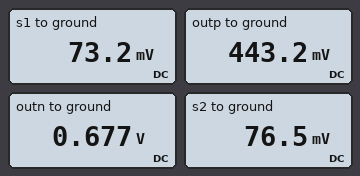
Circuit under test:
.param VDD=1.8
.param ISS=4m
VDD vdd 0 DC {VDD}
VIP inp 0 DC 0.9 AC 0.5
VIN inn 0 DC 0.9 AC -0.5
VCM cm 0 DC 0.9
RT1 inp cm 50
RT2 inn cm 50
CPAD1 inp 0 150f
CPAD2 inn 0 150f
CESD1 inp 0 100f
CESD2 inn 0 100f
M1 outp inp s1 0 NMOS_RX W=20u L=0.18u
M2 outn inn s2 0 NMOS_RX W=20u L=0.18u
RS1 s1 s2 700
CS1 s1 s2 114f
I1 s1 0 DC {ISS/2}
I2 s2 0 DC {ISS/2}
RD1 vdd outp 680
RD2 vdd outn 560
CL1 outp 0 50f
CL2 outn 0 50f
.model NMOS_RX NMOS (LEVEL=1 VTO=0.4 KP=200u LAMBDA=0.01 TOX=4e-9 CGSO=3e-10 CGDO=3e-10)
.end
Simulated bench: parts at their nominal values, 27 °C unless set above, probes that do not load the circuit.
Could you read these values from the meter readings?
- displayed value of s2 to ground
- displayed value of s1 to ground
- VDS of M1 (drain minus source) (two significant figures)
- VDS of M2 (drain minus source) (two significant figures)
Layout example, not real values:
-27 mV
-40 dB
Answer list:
76.5 mV
73.2 mV
370 mV
600 mV
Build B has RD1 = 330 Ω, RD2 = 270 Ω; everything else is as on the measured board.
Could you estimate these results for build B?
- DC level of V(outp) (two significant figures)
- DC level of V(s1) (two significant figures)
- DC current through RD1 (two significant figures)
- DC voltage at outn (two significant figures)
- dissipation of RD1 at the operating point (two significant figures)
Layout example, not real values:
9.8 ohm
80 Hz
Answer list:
1.1 V
78 mV
2.0 mA
1.3 V
1.3 mW
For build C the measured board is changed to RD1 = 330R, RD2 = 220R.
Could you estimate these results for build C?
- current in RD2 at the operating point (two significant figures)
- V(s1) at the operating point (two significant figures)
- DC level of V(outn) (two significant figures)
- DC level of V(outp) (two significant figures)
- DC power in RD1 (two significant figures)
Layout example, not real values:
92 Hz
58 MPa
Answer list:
2.0 mA
78 mV
1.4 V
1.1 V
1.3 mW
